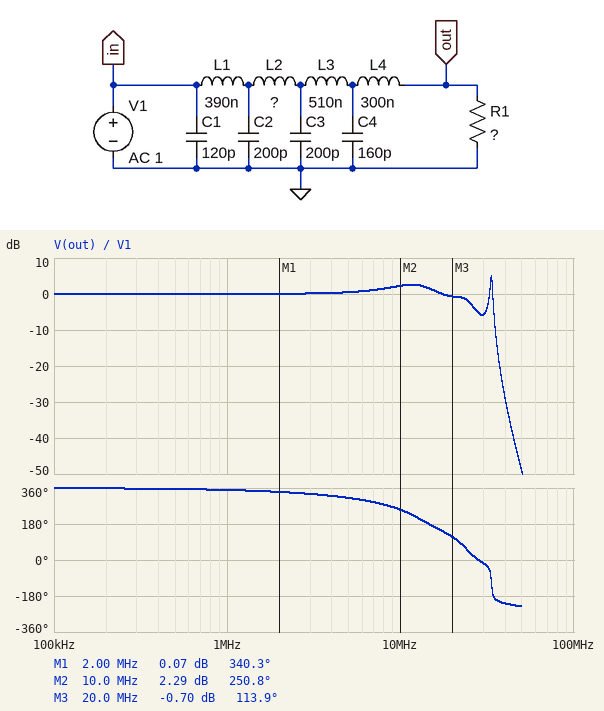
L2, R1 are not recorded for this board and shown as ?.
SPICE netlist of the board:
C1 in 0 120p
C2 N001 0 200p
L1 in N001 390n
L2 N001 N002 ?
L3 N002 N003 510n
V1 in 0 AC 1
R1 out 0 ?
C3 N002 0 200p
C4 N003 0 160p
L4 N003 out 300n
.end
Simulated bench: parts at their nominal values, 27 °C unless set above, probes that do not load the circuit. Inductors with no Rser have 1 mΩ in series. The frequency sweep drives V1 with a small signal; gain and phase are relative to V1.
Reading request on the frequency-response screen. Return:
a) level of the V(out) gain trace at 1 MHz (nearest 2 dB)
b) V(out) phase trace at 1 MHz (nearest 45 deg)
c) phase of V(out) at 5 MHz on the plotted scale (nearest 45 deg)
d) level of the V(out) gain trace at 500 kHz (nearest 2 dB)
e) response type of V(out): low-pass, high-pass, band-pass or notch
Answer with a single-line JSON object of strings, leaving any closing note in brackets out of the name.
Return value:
{"level of the V(out) gain trace at 1 MHz": "0 dB", "V(out) phase trace at 1 MHz": "360 deg", "phase of V(out) at 5 MHz on the plotted scale": "315 deg", "level of the V(out) gain trace at 500 kHz": "0 dB", "response type of V(out): low-pass, high-pass, band-pass or notch": "low-pass"}
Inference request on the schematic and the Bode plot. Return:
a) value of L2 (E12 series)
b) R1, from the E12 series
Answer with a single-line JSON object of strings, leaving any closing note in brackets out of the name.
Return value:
{"value of L2": "330 nH", "R1, from the E12 series": "56 Ω"}
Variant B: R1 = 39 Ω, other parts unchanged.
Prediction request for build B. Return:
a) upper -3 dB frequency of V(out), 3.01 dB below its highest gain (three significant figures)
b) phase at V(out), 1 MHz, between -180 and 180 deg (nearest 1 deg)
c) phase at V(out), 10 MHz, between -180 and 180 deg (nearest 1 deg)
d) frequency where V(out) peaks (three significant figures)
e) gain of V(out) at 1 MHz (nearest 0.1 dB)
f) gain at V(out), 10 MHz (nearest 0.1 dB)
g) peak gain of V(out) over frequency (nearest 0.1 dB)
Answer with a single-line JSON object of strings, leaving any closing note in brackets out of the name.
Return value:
{"upper -3 dB frequency of V(out), 3.01 dB below its highest gain": "34.0 MHz", "phase at V(out), 1 MHz, between -180 and 180 deg": "-14 deg", "phase at V(out), 10 MHz, between -180 and 180 deg": "-104 deg", "frequency where V(out) peaks": "33.5 MHz", "gain of V(out) at 1 MHz": "-0.1 dB", "gain at V(out), 10 MHz": "-0.6 dB", "peak gain of V(out) over frequency": "2.4 dB"}
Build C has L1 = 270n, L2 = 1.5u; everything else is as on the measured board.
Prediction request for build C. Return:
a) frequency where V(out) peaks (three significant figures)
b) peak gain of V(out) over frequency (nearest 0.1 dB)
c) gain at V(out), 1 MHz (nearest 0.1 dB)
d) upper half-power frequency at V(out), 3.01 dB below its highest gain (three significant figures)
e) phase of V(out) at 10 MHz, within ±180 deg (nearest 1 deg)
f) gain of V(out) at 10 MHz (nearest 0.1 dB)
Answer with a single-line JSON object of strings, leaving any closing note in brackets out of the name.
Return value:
{"frequency where V(out) peaks": "23.8 MHz", "peak gain of V(out) over frequency": "15.6 dB", "gain at V(out), 1 MHz": "-0.1 dB", "upper half-power frequency at V(out), 3.01 dB below its highest gain": "24.1 MHz", "phase of V(out) at 10 MHz, within ±180 deg": "-138 deg", "gain of V(out) at 10 MHz": "-3.8 dB"}
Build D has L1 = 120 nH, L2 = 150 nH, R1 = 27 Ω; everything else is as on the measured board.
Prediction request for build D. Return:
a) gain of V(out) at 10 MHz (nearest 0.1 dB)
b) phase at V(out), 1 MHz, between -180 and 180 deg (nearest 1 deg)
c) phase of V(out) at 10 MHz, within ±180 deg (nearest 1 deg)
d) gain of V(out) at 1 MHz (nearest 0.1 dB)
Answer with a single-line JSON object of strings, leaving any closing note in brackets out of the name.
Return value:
{"gain of V(out) at 10 MHz": "-4.5 dB", "phase at V(out), 1 MHz, between -180 and 180 deg": "-14 deg", "phase of V(out) at 10 MHz, within ±180 deg": "-79 deg", "gain of V(out) at 1 MHz": "-0.2 dB"}
